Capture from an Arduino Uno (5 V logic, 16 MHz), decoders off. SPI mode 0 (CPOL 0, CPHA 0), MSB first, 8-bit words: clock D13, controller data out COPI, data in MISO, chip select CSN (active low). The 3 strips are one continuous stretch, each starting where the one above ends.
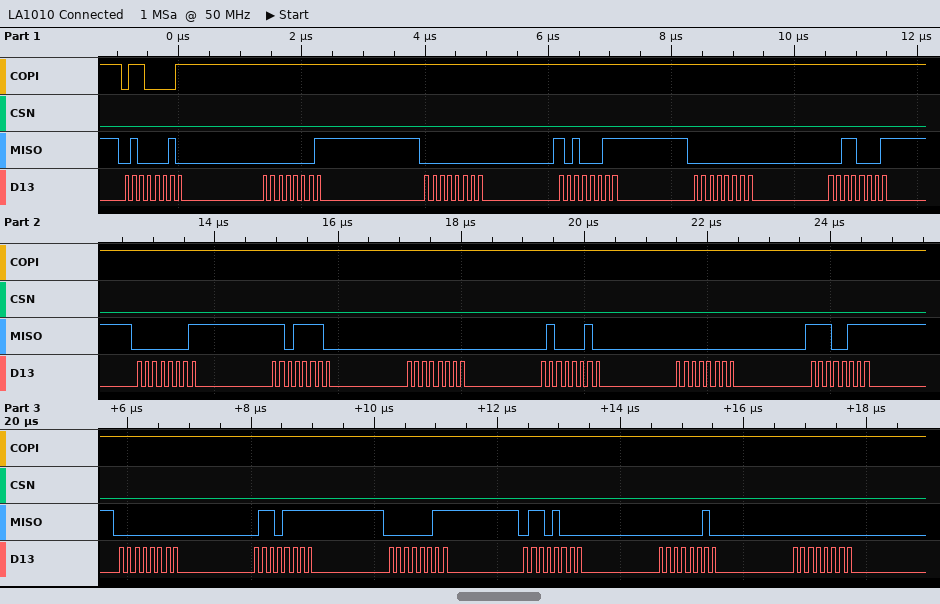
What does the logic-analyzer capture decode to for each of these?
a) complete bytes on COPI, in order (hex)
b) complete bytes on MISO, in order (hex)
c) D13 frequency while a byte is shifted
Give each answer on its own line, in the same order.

0x61 0xFF 0xFF 0xFF 0xFF 0xFF 0xFF 0xFF 0xFF 0xFF 0xFF 0xFF 0xFF 0xFF 0xFF 0xFF 0xFF 0xFF
0x42 0x01 0x00 0xA3 0x00 0x31 0x01 0xDE 0x00 0x42 0x00 0xE7 0x00 0x6F 0x03 0x68 0x02 0x00
8 MHz
